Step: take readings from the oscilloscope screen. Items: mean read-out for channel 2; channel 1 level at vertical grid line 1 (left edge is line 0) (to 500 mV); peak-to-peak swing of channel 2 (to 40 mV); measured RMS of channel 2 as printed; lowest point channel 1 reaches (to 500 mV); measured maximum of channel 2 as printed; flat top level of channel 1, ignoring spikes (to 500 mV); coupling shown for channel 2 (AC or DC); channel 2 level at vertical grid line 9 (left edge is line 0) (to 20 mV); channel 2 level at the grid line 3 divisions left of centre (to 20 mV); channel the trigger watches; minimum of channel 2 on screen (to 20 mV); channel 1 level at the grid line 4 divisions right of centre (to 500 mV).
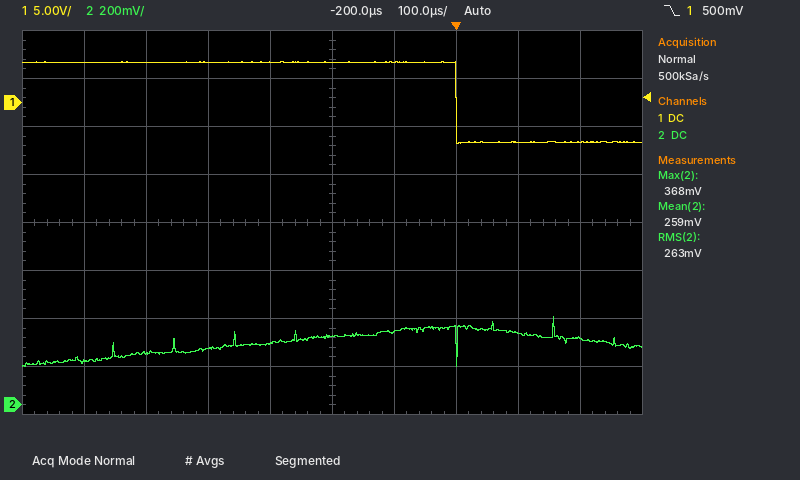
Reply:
259 mV
4.0 V
200 mV
263 mV
-4.5 V
368 mV
4.0 V
DC
280 mV
220 mV
channel 1
160 mV
-4.0 V
